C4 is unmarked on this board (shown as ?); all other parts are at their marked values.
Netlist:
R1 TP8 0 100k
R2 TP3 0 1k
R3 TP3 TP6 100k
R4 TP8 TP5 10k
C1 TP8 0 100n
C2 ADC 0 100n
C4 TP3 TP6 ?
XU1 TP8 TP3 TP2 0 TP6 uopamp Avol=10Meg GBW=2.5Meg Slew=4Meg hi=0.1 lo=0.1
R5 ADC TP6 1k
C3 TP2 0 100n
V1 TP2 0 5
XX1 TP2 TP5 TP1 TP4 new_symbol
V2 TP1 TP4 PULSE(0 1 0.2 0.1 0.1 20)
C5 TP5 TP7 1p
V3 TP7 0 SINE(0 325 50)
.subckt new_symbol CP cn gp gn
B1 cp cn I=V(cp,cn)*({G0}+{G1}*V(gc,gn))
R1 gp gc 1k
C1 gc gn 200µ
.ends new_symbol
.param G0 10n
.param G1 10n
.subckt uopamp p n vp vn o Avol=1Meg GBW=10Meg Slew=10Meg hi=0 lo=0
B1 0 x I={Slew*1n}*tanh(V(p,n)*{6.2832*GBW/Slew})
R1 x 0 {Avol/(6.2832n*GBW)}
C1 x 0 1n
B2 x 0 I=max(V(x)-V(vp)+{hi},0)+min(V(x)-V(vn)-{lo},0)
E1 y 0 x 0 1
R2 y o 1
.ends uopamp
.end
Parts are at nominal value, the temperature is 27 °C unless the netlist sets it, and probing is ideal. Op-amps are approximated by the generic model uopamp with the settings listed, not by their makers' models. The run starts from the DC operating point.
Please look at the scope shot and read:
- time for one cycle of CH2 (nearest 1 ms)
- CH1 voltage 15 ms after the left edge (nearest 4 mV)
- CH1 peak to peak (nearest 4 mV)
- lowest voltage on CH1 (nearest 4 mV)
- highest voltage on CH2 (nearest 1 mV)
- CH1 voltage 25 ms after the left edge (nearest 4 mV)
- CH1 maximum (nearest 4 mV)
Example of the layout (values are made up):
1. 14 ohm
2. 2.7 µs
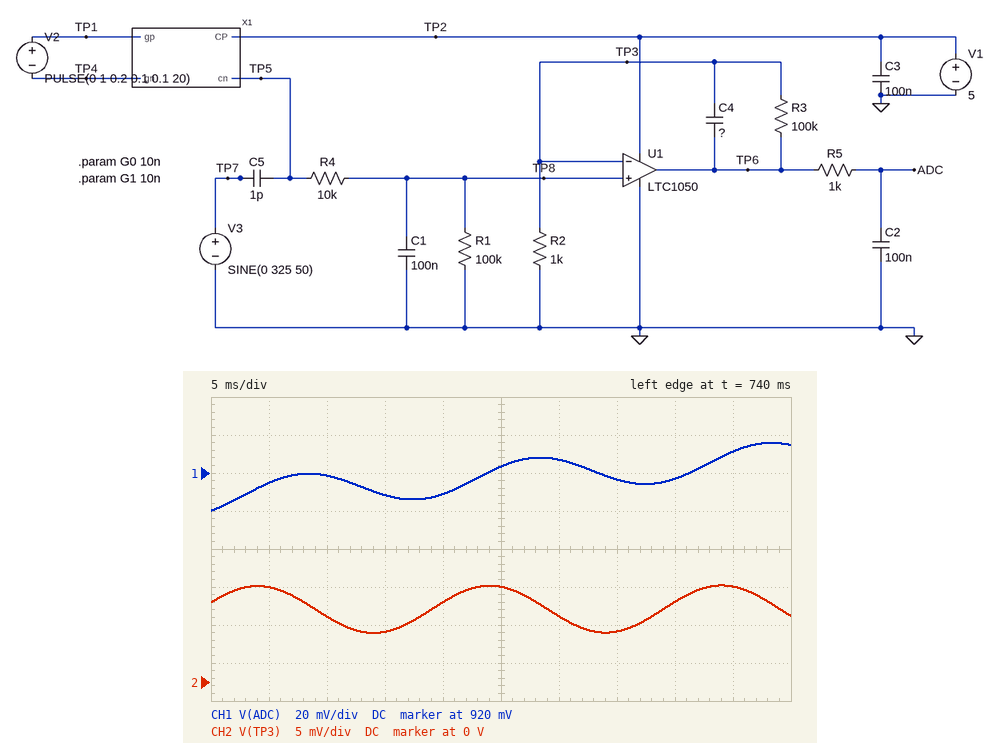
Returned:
1. 20 ms
2. 908 mV
3. 36 mV
4. 900 mV
5. 13 mV
6. 924 mV
7. 936 mV
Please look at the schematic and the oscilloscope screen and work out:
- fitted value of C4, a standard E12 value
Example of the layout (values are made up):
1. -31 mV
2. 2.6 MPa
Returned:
1. 1.2 µF
